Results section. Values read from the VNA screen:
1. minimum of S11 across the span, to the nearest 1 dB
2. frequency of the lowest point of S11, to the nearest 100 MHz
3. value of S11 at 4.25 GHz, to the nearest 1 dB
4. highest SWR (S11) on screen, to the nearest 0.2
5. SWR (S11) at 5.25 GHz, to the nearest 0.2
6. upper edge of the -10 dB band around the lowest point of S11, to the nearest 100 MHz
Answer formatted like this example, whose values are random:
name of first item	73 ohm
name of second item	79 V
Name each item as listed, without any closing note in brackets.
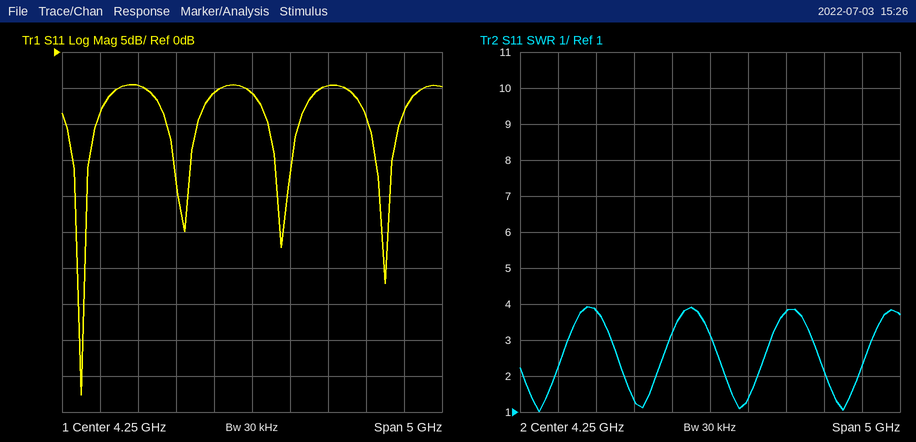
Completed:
minimum of S11 across the span, to the nearest 1 dB	-48 dB
frequency of the lowest point of S11, to the nearest 100 MHz	2.0 GHz
value of S11 at 4.25 GHz, to the nearest 1 dB	-6 dB
highest SWR (S11) on screen, to the nearest 0.2	4.0
SWR (S11) at 5.25 GHz, to the nearest 0.2	3.8
upper edge of the -10 dB band around the lowest point of S11, to the nearest 100 MHz	2.2 GHz
